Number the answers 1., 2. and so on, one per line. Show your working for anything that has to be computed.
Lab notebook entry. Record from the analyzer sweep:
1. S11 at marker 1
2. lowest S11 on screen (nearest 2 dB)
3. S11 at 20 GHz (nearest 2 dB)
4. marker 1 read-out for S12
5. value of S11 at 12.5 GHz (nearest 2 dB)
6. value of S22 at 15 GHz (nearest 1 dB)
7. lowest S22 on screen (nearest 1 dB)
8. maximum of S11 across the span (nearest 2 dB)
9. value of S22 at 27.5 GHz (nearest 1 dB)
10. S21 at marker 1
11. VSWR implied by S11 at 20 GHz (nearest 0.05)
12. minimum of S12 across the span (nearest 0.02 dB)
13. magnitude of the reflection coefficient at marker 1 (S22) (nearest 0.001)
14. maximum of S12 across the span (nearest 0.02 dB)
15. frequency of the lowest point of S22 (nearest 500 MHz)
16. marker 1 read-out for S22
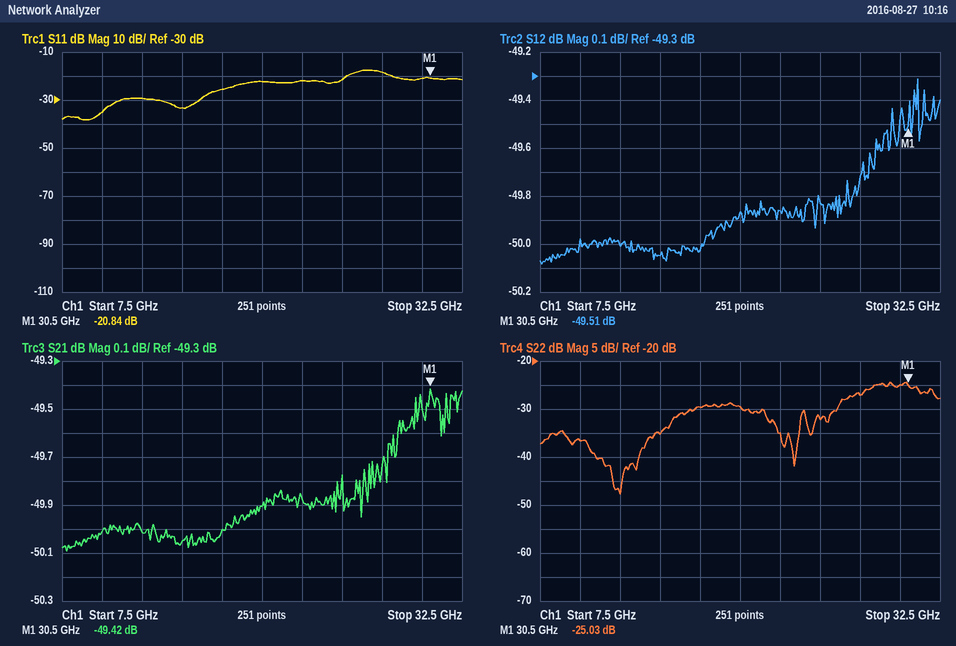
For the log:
1. -20.84 dB
2. -38 dB
3. -22 dB
4. -49.51 dB
5. -30 dB
6. -35 dB
7. -48 dB
8. -18 dB
9. -27 dB
10. -49.42 dB
11. |Γ| = 10^(-22/20) = 0.0794; VSWR = (1 + 0.0794)/(1 − 0.0794) ≈ 1.17, so 1.15 to the nearest 0.05
12. -50.08 dB
13. 10^(-25.03/20) ≈ 0.056
14. -49.32 dB
15. 12.5 GHz
16. -25.03 dB
